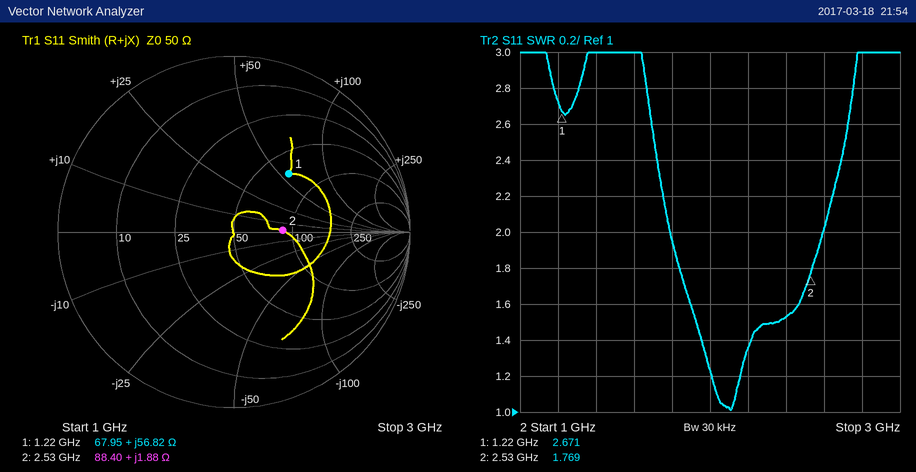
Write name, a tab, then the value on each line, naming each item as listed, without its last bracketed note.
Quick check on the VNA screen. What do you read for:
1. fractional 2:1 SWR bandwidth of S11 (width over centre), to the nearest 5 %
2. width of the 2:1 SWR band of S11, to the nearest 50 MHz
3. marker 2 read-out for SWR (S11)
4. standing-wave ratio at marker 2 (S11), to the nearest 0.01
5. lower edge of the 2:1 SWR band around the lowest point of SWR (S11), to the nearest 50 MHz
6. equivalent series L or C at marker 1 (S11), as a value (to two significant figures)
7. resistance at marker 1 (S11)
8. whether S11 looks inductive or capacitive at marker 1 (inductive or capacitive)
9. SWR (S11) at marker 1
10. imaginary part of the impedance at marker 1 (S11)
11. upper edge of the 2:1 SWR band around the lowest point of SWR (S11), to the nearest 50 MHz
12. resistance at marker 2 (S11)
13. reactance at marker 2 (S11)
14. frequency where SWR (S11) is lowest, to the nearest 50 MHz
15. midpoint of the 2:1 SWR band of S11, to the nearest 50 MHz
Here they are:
fractional 2:1 SWR bandwidth of S11 (width over centre), to the nearest 5 %	35 %
width of the 2:1 SWR band of S11, to the nearest 50 MHz	800 MHz
marker 2 read-out for SWR	1.769
standing-wave ratio at marker 2 (S11), to the nearest 0.01	1.77
lower edge of the 2:1 SWR band around the lowest point of SWR (S11), to the nearest 50 MHz	1.80 GHz
equivalent series L or C at marker 1 (S11), as a value	7.4 nH
resistance at marker 1	67.95 Ω
whether S11 looks inductive or capacitive at marker 1	inductive
SWR (S11) at marker 1	2.671
imaginary part of the impedance at marker 1	+56.82 Ω
upper edge of the 2:1 SWR band around the lowest point of SWR (S11), to the nearest 50 MHz	2.60 GHz
resistance at marker 2	88.40 Ω
reactance at marker 2	+1.88 Ω
frequency where SWR (S11) is lowest, to the nearest 50 MHz	2.10 GHz
midpoint of the 2:1 SWR band of S11, to the nearest 50 MHz	2.20 GHz
